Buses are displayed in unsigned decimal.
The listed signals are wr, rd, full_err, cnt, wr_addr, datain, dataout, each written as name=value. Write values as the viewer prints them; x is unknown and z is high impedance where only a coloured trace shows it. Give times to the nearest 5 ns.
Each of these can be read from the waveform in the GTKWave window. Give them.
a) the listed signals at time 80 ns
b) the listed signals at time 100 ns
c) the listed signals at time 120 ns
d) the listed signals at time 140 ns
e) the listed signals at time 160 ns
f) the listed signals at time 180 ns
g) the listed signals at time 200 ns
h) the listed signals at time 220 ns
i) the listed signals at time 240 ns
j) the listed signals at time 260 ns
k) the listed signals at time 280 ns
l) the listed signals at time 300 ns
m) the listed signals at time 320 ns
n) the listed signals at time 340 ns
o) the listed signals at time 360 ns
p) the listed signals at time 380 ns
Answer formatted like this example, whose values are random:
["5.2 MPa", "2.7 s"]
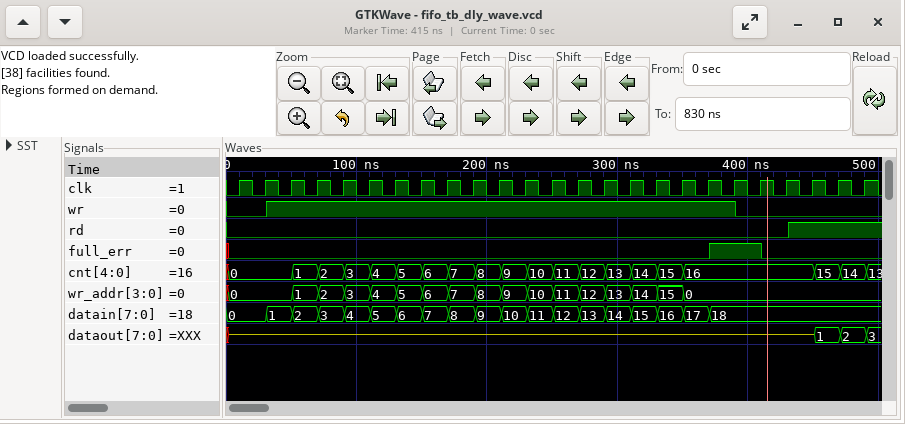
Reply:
["wr=1, rd=0, full_err=0, cnt=2, wr_addr=2, datain=3, dataout=z", "wr=1, rd=0, full_err=0, cnt=3, wr_addr=3, datain=4, dataout=z", "wr=1, rd=0, full_err=0, cnt=4, wr_addr=4, datain=5, dataout=z", "wr=1, rd=0, full_err=0, cnt=5, wr_addr=5, datain=6, dataout=z", "wr=1, rd=0, full_err=0, cnt=6, wr_addr=6, datain=7, dataout=z", "wr=1, rd=0, full_err=0, cnt=7, wr_addr=7, datain=8, dataout=z", "wr=1, rd=0, full_err=0, cnt=8, wr_addr=8, datain=9, dataout=z", "wr=1, rd=0, full_err=0, cnt=9, wr_addr=9, datain=10, dataout=z", "wr=1, rd=0, full_err=0, cnt=10, wr_addr=10, datain=11, dataout=z", "wr=1, rd=0, full_err=0, cnt=11, wr_addr=11, datain=12, dataout=z", "wr=1, rd=0, full_err=0, cnt=12, wr_addr=12, datain=13, dataout=z", "wr=1, rd=0, full_err=0, cnt=13, wr_addr=13, datain=14, dataout=z", "wr=1, rd=0, full_err=0, cnt=14, wr_addr=14, datain=15, dataout=z", "wr=1, rd=0, full_err=0, cnt=15, wr_addr=15, datain=16, dataout=z", "wr=1, rd=0, full_err=0, cnt=16, wr_addr=0, datain=17, dataout=z", "wr=1, rd=0, full_err=1, cnt=16, wr_addr=0, datain=18, dataout=z"]
